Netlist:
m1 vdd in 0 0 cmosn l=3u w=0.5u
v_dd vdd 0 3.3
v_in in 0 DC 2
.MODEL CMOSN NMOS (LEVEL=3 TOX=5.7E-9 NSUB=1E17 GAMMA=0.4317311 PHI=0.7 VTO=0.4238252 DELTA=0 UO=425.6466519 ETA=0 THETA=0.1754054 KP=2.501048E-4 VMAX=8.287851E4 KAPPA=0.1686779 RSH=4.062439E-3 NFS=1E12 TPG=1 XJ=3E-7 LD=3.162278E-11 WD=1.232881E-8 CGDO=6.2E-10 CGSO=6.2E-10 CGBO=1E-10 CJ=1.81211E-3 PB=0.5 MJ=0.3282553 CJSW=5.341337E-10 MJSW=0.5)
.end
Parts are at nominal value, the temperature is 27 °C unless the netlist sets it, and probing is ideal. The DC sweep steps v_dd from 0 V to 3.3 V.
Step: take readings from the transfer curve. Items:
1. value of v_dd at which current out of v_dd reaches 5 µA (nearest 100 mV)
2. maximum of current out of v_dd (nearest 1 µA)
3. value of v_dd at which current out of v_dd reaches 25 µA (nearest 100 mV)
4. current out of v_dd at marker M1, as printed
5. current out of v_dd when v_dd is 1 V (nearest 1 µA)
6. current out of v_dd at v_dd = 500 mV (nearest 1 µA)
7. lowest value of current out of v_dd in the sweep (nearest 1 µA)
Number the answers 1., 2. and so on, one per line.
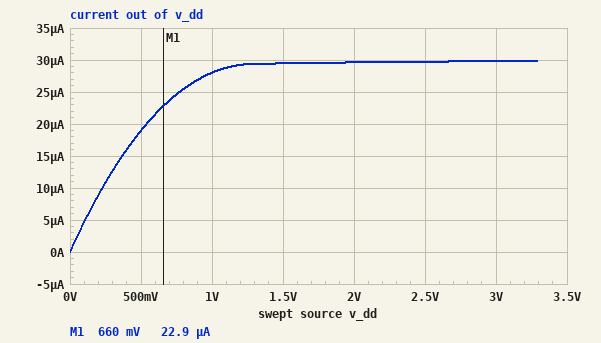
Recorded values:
1. 100 mV
2. 30 µA
3. 800 mV
4. 22.9 µA
5. 28 µA
6. 19 µA
7. 0 A
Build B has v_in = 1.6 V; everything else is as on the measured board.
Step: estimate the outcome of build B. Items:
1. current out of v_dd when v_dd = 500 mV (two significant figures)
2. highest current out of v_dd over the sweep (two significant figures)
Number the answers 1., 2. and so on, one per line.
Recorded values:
1. 14 µA
2. 18 µA
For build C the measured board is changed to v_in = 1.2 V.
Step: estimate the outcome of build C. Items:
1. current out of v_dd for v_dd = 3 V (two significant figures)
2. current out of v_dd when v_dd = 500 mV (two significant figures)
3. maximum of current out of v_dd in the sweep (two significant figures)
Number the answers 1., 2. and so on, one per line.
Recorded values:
1. 8.8 µA
2. 8.2 µA
3. 8.9 µA
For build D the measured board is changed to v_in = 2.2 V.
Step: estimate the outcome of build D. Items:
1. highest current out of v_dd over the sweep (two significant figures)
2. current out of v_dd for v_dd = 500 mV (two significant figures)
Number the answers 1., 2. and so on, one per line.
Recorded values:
1. 36 µA
2. 21 µA
